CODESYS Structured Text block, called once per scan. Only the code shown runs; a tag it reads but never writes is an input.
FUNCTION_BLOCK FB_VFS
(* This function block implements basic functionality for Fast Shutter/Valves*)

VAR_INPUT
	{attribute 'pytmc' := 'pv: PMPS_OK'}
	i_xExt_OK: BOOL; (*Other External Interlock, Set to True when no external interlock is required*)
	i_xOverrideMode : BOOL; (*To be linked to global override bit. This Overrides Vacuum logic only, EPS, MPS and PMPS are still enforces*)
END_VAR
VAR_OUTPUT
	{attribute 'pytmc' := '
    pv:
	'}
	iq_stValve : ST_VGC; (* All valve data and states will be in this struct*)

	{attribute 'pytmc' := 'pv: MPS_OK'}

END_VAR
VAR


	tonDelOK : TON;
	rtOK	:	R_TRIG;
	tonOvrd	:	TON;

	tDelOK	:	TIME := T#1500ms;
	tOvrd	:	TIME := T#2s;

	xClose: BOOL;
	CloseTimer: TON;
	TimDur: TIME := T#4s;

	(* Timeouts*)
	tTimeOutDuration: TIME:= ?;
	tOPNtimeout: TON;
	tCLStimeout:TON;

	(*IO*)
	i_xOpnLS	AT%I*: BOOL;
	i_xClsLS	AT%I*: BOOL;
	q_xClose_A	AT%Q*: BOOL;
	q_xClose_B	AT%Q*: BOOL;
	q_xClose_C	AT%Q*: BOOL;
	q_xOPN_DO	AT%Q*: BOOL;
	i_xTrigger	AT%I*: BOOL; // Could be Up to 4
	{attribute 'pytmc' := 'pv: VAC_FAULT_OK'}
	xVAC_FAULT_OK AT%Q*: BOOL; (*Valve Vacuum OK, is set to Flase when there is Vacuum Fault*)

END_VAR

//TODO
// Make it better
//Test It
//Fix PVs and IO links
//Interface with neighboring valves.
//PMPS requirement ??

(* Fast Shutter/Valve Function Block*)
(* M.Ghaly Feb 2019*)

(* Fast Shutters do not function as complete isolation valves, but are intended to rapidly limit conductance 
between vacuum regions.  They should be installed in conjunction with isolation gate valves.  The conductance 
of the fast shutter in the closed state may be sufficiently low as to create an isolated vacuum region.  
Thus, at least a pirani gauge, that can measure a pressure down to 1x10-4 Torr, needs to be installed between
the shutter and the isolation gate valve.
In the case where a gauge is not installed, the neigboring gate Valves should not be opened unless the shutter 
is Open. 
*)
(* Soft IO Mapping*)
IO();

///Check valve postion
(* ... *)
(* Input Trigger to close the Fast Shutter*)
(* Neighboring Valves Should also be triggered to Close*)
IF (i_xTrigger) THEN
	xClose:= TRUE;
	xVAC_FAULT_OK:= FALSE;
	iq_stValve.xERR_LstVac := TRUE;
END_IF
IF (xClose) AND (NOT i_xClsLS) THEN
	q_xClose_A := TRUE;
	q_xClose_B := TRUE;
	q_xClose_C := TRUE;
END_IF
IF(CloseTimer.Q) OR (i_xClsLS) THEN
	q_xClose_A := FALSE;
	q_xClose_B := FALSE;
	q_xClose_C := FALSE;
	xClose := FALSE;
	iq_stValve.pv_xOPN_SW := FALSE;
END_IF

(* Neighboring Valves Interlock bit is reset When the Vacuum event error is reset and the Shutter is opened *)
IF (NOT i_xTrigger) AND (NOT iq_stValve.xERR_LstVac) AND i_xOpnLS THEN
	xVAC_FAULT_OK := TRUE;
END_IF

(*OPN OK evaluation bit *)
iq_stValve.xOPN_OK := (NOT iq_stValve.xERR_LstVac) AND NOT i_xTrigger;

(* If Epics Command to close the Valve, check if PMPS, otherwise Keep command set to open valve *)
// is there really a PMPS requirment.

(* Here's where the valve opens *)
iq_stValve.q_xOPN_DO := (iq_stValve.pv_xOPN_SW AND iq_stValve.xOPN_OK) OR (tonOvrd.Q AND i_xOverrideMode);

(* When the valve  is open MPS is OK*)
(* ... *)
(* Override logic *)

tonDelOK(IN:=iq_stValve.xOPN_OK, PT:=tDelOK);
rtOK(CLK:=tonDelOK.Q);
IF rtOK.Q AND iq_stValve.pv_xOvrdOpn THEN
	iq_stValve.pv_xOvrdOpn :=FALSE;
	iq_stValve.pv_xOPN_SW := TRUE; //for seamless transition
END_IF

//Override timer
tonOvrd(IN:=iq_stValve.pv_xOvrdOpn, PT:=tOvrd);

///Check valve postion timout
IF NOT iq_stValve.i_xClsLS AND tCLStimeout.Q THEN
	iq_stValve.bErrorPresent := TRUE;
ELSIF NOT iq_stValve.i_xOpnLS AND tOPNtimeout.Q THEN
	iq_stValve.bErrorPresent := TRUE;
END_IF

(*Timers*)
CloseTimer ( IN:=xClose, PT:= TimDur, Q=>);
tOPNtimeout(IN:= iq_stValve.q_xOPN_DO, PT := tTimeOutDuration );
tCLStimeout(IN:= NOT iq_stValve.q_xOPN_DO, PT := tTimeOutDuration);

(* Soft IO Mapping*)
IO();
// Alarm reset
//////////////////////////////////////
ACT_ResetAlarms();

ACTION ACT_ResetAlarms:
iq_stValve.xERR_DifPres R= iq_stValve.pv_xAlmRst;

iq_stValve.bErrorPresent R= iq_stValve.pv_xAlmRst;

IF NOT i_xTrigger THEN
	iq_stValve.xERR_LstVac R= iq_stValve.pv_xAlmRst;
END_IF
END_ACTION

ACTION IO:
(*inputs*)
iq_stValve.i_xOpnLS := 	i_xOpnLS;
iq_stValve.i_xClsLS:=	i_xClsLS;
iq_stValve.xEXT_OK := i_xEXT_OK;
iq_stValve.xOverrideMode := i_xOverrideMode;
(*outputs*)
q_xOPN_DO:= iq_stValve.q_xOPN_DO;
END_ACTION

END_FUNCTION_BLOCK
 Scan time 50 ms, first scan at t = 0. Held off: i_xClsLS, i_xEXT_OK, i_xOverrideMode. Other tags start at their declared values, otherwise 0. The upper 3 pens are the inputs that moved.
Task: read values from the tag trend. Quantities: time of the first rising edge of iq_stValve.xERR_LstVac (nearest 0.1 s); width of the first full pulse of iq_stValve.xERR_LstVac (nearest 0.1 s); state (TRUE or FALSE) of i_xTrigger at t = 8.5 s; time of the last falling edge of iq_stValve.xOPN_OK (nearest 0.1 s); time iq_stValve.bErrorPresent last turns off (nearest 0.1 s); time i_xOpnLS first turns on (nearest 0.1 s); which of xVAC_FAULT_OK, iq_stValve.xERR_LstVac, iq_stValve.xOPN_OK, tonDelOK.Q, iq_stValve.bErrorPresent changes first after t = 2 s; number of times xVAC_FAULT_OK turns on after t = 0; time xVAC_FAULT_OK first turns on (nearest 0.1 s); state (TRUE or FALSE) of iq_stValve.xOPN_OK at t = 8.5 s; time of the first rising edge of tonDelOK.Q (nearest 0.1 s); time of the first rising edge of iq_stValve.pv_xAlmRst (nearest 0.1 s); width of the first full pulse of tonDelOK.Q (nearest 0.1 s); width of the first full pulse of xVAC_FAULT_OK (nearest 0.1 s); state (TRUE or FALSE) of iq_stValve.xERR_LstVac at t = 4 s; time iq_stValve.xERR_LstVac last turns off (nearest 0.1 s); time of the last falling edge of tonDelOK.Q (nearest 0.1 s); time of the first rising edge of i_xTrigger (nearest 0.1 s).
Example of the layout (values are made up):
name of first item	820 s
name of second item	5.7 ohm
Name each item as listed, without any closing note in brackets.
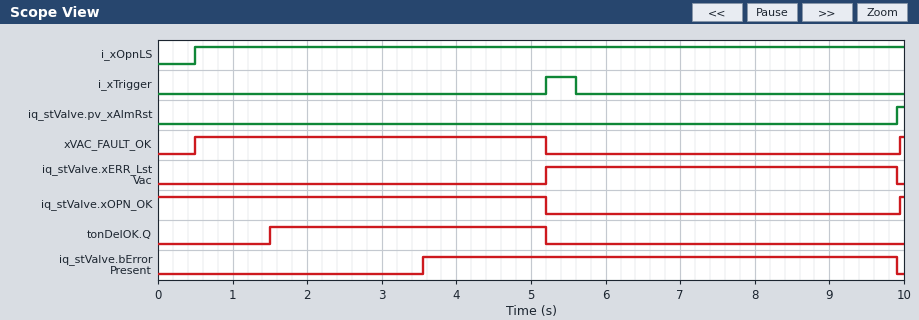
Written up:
time of the first rising edge of iq_stValve.xERR_LstVac	5.2 s
width of the first full pulse of iq_stValve.xERR_LstVac	4.7 s
state (TRUE or FALSE) of i_xTrigger at t = 8.5 s	FALSE
time of the last falling edge of iq_stValve.xOPN_OK	5.2 s
time iq_stValve.bErrorPresent last turns off	9.9 s
time i_xOpnLS first turns on	0.5 s
which of xVAC_FAULT_OK, iq_stValve.xERR_LstVac, iq_stValve.xOPN_OK, tonDelOK.Q, iq_stValve.bErrorPresent changes first after t = 2 s	iq_stValve.bErrorPresent
number of times xVAC_FAULT_OK turns on after t = 0	2
time xVAC_FAULT_OK first turns on	0.5 s
state (TRUE or FALSE) of iq_stValve.xOPN_OK at t = 8.5 s	FALSE
time of the first rising edge of tonDelOK.Q	1.5 s
time of the first rising edge of iq_stValve.pv_xAlmRst	9.9 s
width of the first full pulse of tonDelOK.Q	3.7 s
width of the first full pulse of xVAC_FAULT_OK	4.7 s
state (TRUE or FALSE) of iq_stValve.xERR_LstVac at t = 4 s	FALSE
time iq_stValve.xERR_LstVac last turns off	9.9 s
time of the last falling edge of tonDelOK.Q	5.2 s
time of the first rising edge of i_xTrigger	5.2 s
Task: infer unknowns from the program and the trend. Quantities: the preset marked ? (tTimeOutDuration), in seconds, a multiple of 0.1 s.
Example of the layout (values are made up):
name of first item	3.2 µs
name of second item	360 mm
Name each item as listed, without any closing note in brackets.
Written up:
the preset marked ? (tTimeOutDuration), in seconds, a multiple of 0.1 s	3.5 s
